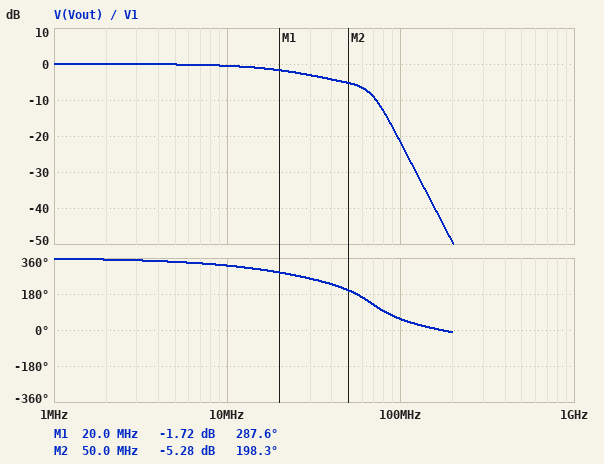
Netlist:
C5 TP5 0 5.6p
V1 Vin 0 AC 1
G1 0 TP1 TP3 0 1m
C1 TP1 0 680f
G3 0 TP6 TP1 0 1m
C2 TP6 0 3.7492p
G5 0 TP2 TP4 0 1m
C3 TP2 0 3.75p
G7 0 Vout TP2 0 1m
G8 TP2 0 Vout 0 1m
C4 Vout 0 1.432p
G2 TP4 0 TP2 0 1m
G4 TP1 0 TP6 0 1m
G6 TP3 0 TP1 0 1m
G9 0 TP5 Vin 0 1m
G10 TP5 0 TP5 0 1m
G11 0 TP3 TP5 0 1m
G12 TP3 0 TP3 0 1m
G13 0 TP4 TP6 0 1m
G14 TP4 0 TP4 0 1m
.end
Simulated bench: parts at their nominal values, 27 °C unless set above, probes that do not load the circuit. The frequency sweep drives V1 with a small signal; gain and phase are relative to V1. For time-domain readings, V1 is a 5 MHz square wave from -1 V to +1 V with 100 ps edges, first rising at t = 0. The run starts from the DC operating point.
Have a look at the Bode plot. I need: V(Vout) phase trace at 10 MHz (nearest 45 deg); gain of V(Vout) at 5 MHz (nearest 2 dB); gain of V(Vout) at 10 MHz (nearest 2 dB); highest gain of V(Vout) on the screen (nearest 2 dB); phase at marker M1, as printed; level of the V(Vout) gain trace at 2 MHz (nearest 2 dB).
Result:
315 deg
0 dB
0 dB
0 dB
287.6 deg
0 dB
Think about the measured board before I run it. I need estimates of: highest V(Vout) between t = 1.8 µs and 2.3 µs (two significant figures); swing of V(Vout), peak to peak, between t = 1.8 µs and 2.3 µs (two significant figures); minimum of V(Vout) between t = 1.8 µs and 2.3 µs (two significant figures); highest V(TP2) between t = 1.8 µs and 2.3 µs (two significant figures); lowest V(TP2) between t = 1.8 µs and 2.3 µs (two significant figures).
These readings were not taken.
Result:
1.0 V
2.0 V
-1.0 V
310 mV
-310 mV
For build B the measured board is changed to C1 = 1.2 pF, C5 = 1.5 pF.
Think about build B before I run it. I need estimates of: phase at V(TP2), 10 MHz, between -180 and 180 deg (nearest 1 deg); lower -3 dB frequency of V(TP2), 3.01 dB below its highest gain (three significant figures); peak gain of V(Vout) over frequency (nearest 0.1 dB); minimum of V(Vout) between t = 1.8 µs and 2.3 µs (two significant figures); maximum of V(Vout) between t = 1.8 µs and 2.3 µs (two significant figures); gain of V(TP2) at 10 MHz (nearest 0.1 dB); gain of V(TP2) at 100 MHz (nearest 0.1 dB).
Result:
66 deg
40.9 MHz
0.6 dB
-1.3 V
1.3 V
-20.9 dB
-14.7 dB
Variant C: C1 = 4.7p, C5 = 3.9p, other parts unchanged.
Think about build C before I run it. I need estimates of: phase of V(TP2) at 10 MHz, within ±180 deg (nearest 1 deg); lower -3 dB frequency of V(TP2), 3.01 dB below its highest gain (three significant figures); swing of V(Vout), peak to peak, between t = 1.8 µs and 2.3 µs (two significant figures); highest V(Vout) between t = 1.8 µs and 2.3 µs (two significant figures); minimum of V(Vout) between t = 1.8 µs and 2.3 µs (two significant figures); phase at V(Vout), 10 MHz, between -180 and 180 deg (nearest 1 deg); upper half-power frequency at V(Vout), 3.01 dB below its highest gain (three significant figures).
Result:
57 deg
24.5 MHz
2.8 V
1.4 V
-1.4 V
-33 deg
45.3 MHz
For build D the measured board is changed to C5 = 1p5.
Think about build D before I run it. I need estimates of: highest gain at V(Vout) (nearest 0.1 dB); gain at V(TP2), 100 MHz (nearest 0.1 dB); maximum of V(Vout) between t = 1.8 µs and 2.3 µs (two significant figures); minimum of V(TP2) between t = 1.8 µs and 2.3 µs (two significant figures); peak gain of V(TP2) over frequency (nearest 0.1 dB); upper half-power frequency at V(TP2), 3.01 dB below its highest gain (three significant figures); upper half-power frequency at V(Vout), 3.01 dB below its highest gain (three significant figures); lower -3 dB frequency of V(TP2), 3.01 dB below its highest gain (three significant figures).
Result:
0 dB
-14.3 dB
1.2 V
-480 mV
-5.7 dB
80.6 MHz
72.4 MHz
41.2 MHz
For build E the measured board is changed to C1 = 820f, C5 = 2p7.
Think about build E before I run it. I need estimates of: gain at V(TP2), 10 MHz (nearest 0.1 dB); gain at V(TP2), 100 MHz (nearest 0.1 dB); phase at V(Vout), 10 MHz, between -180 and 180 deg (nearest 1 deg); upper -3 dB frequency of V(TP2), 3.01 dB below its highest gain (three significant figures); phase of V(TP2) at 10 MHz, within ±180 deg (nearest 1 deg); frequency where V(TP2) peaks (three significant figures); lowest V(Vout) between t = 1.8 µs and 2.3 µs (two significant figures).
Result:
-21.0 dB
-17.4 dB
-28 deg
78.2 MHz
62 deg
60.3 MHz
-1.1 V
